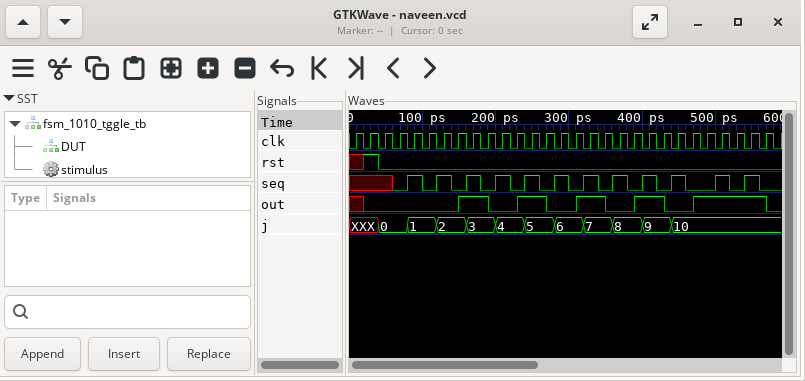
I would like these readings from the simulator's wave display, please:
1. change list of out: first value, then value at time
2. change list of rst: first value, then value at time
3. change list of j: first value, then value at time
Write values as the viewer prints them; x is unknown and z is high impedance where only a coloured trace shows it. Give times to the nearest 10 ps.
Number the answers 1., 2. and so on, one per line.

1. x, 0 at 20 ps, 1 at 150 ps, 0 at 190 ps, 1 at 230 ps, 0 at 270 ps, 1 at 310 ps, 0 at 350 ps, 1 at 390 ps, 0 at 430 ps, 1 at 470 ps, 0 at 570 ps
2. x, 1 at 20 ps, 0 at 40 ps
3. XXX, 0 at 40 ps, 1 at 80 ps, 2 at 120 ps, 3 at 160 ps, 4 at 200 ps, 5 at 240 ps, 6 at 280 ps, 7 at 320 ps, 8 at 360 ps, 9 at 400 ps, 10 at 440 ps
